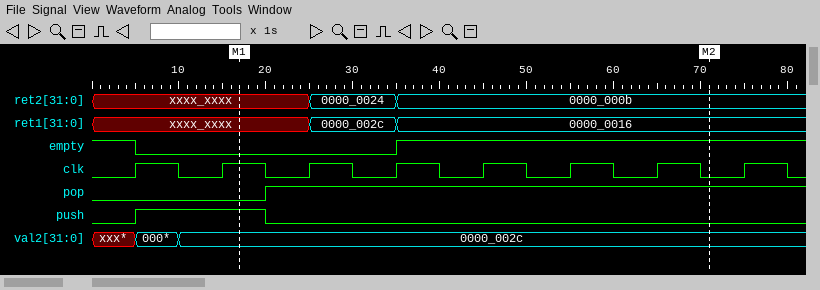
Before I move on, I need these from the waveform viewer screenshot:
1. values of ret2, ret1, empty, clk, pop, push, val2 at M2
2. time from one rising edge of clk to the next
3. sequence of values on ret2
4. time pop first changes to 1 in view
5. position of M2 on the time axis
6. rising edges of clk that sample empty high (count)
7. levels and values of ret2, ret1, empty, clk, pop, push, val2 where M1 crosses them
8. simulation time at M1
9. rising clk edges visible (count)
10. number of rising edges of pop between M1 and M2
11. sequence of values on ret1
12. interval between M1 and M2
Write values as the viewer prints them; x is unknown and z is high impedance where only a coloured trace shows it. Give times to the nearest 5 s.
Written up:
ret2=0000_000b, ret1=0000_0016, empty=1, clk=0, pop=1, push=0, val2=0000_002c
10 s
xxxx_xxxx, 0000_0024, 0000_000b
20 s
70 s
5
ret2=xxxx_xxxx, ret1=xxxx_xxxx, empty=0, clk=1, pop=0, push=1, val2=0000_002c
15 s
8
1
xxxx_xxxx, 0000_002c, 0000_0016
55 s
